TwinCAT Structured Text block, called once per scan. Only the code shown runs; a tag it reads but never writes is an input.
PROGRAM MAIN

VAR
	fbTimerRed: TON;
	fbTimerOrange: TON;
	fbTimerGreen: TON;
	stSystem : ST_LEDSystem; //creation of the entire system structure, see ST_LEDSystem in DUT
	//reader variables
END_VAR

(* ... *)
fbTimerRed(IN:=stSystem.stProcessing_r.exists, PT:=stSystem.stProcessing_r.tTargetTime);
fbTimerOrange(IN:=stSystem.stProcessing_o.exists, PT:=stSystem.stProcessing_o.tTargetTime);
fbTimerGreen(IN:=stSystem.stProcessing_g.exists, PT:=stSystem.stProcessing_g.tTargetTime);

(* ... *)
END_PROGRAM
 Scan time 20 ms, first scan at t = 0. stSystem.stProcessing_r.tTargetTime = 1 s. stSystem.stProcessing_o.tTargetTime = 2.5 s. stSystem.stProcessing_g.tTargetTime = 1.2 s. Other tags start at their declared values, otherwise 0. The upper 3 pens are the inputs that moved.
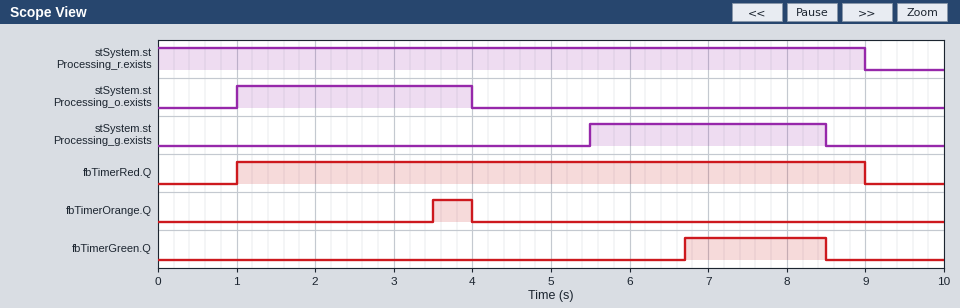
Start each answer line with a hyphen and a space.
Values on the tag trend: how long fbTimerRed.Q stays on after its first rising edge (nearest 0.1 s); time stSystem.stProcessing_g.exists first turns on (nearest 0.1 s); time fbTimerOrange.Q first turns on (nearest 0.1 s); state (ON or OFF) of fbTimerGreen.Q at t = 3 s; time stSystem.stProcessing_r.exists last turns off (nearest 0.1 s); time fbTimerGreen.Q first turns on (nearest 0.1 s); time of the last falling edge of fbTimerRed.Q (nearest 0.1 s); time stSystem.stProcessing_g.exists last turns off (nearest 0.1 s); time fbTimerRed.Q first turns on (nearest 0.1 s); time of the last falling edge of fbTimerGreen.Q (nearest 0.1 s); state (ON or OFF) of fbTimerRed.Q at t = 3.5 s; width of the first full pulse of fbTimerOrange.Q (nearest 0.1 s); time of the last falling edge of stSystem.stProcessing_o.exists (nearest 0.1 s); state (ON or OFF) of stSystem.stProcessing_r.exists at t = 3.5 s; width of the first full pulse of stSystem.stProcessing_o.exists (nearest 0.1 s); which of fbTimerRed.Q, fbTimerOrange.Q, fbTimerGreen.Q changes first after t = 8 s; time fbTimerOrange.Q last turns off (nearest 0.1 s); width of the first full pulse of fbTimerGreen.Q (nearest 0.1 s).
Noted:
- 8.0 s
- 5.5 s
- 3.5 s
- OFF
- 9.0 s
- 6.7 s
- 9.0 s
- 8.5 s
- 1.0 s
- 8.5 s
- ON
- 0.5 s
- 4.0 s
- ON
- 3.0 s
- fbTimerGreen.Q
- 4.0 s
- 1.8 s
